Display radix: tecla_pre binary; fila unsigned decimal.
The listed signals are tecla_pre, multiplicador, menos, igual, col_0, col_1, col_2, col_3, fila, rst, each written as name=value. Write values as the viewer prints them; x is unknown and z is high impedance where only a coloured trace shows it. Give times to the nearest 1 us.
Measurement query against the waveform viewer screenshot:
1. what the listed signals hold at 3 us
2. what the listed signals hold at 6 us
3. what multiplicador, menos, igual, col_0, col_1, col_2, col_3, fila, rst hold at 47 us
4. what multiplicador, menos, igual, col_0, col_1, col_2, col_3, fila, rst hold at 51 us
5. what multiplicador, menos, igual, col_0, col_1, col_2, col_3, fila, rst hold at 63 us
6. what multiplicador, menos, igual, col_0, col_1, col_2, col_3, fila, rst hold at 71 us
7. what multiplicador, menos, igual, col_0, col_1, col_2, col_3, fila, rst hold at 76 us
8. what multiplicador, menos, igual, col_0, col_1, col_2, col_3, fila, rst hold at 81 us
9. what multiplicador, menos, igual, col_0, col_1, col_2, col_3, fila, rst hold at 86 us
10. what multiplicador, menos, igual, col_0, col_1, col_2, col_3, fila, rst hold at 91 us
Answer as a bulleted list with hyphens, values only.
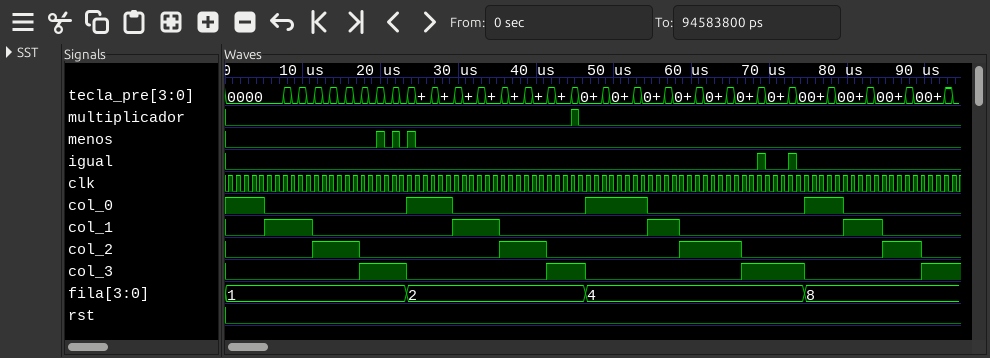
- tecla_pre=0000, multiplicador=0, menos=0, igual=0, col_0=1, col_1=0, col_2=0, col_3=0, fila=1, rst=0
- tecla_pre=0000, multiplicador=0, menos=0, igual=0, col_0=0, col_1=1, col_2=0, col_3=0, fila=1, rst=0
- multiplicador=0, menos=0, igual=0, col_0=1, col_1=0, col_2=0, col_3=0, fila=4, rst=0
- multiplicador=0, menos=0, igual=0, col_0=1, col_1=0, col_2=0, col_3=0, fila=4, rst=0
- multiplicador=0, menos=0, igual=0, col_0=0, col_1=0, col_2=1, col_3=0, fila=4, rst=0
- multiplicador=0, menos=0, igual=0, col_0=0, col_1=0, col_2=0, col_3=1, fila=4, rst=0
- multiplicador=0, menos=0, igual=0, col_0=1, col_1=0, col_2=0, col_3=0, fila=8, rst=0
- multiplicador=0, menos=0, igual=0, col_0=0, col_1=1, col_2=0, col_3=0, fila=8, rst=0
- multiplicador=0, menos=0, igual=0, col_0=0, col_1=0, col_2=1, col_3=0, fila=8, rst=0
- multiplicador=0, menos=0, igual=0, col_0=0, col_1=0, col_2=0, col_3=1, fila=8, rst=0
